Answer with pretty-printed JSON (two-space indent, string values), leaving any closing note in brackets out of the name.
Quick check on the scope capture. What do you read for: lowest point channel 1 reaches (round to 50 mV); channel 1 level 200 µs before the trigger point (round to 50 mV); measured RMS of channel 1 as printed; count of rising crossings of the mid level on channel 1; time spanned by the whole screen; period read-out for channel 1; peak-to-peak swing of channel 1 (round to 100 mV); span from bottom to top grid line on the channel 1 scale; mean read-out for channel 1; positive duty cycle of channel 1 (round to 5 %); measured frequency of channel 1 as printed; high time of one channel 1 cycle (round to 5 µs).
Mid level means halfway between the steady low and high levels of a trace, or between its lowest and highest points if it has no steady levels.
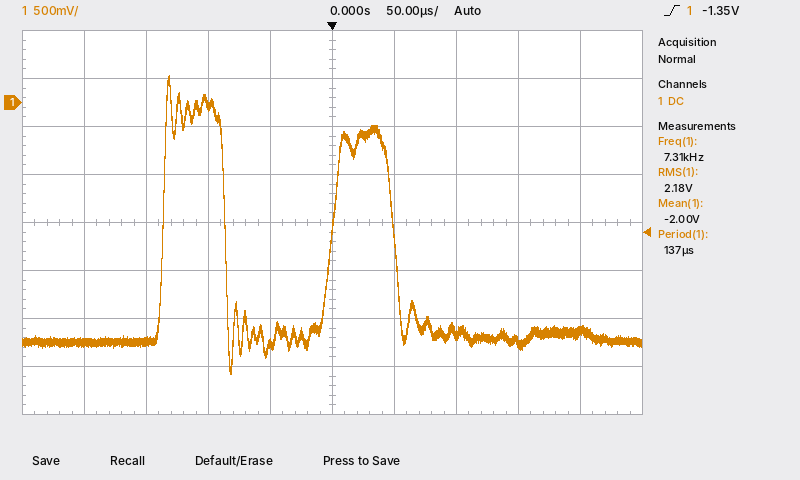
{
  "lowest point channel 1 reaches": "-2.85 V",
  "channel 1 level 200 µs before the trigger point": "-2.50 V",
  "measured RMS of channel 1 as printed": "2.18 V",
  "count of rising crossings of the mid level on channel 1": "2",
  "time spanned by the whole screen": "500 µs",
  "period read-out for channel 1": "137 µs",
  "peak-to-peak swing of channel 1": "3.10 V",
  "span from bottom to top grid line on the channel 1 scale": "4 V",
  "mean read-out for channel 1": "-2.00 V",
  "positive duty cycle of channel 1": "35 %",
  "measured frequency of channel 1 as printed": "7.31 kHz",
  "high time of one channel 1 cycle": "50 µs"
}
